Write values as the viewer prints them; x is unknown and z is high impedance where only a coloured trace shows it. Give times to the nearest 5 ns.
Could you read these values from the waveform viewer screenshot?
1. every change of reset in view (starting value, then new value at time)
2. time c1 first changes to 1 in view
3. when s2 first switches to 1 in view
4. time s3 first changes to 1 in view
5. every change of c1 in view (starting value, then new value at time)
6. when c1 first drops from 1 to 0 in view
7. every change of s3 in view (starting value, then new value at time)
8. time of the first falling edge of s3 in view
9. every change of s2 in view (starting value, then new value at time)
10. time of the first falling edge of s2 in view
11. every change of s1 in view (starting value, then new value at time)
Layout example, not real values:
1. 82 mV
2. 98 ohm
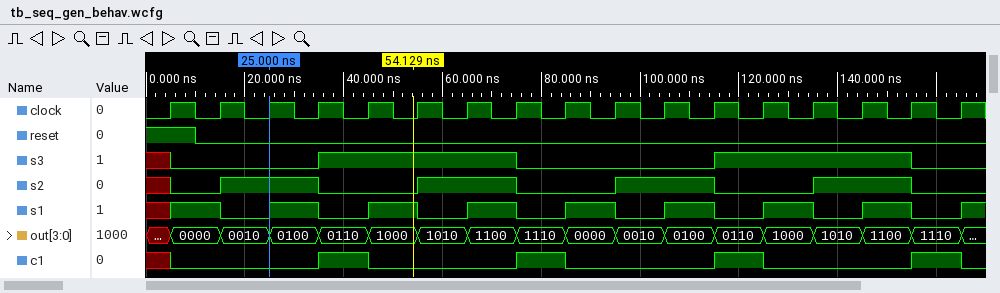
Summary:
1. 1, 0 at 10 ns
2. 35 ns
3. 15 ns
4. 35 ns
5. x, 0 at 5 ns, 1 at 35 ns, 0 at 45 ns, 1 at 75 ns, 0 at 85 ns, 1 at 115 ns, 0 at 125 ns, 1 at 155 ns, 0 at 165 ns
6. 45 ns
7. x, 0 at 5 ns, 1 at 35 ns, 0 at 75 ns, 1 at 115 ns, 0 at 155 ns
8. 75 ns
9. x, 0 at 5 ns, 1 at 15 ns, 0 at 35 ns, 1 at 55 ns, 0 at 75 ns, 1 at 95 ns, 0 at 115 ns, 1 at 135 ns, 0 at 155 ns
10. 35 ns
11. x, 1 at 5 ns, 0 at 15 ns, 1 at 25 ns, 0 at 35 ns, 1 at 45 ns, 0 at 55 ns, 1 at 65 ns, 0 at 75 ns, 1 at 85 ns, 0 at 95 ns, 1 at 105 ns, 0 at 115 ns, 1 at 125 ns, 0 at 135 ns, 1 at 145 ns, 0 at 155 ns, 1 at 165 ns
